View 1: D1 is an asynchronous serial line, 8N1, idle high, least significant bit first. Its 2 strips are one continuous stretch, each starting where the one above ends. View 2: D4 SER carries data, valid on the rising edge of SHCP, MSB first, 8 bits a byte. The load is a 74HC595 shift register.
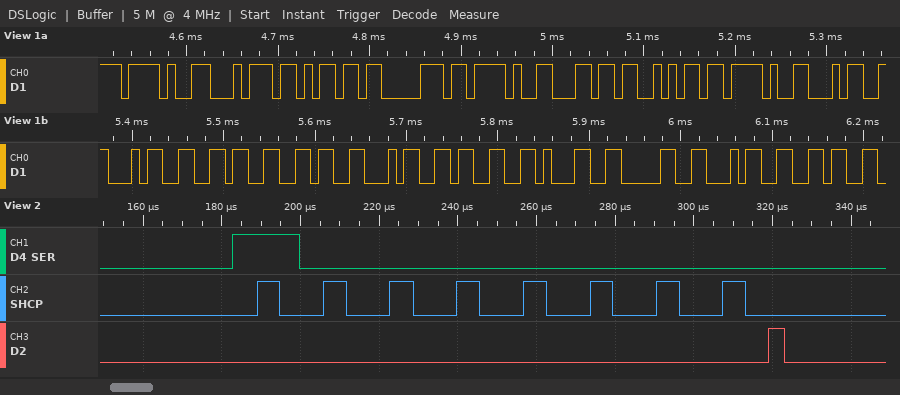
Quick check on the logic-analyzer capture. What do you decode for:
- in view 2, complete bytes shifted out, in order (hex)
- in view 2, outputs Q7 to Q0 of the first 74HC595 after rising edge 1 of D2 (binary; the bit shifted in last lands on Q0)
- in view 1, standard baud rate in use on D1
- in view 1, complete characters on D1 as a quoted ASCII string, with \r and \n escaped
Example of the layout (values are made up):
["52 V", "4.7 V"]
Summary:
["80", "10000000", "115200 baud", "\"/tmp/lj/4466431046\""]
